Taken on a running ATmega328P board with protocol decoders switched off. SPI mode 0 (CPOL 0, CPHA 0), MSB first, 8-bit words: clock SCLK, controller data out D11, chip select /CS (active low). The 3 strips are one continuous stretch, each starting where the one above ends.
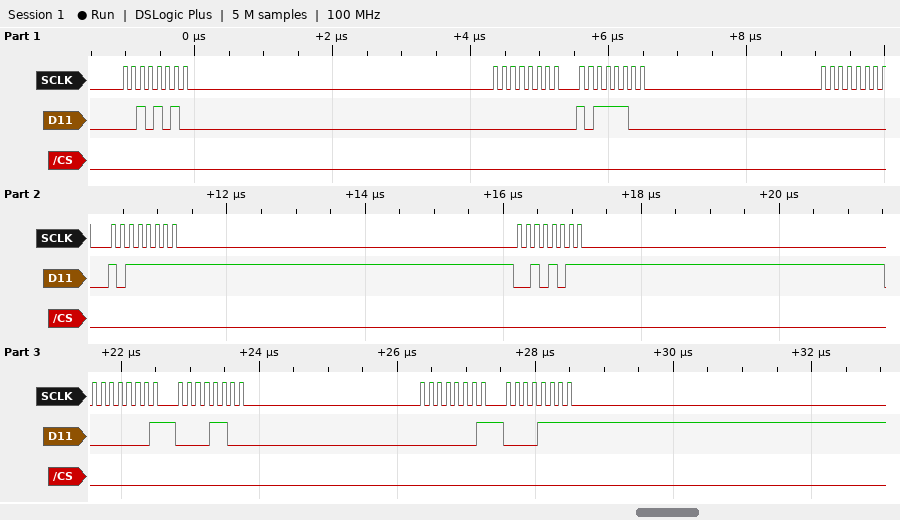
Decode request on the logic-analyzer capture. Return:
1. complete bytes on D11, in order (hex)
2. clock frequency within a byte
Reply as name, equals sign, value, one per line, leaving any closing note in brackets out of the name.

complete bytes on D11, in order = 2A 00 BC 00 BF 2B 01 0C 01 0F
clock frequency within a byte = 8 MHz
